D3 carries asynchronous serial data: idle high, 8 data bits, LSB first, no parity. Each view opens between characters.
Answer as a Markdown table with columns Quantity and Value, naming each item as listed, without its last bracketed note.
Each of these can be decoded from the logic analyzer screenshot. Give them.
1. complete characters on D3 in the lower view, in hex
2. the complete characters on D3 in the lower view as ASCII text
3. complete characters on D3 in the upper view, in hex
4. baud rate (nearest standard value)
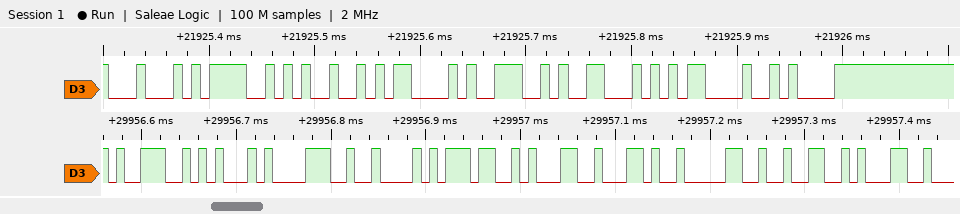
| Quantity | Value |
|---|---|
| complete characters on D3 in the lower view, in hex | 39, 45, 38, 42, 37, 31, 2C, 30, 32, 31 |
| the complete characters on D3 in the lower view as ASCII text | "9E8B71,021" |
| complete characters on D3 in the upper view, in hex | 44, 4F, 49, 43, 4E, 46, 0D, 0A |
| baud rate | 115200 baud |
